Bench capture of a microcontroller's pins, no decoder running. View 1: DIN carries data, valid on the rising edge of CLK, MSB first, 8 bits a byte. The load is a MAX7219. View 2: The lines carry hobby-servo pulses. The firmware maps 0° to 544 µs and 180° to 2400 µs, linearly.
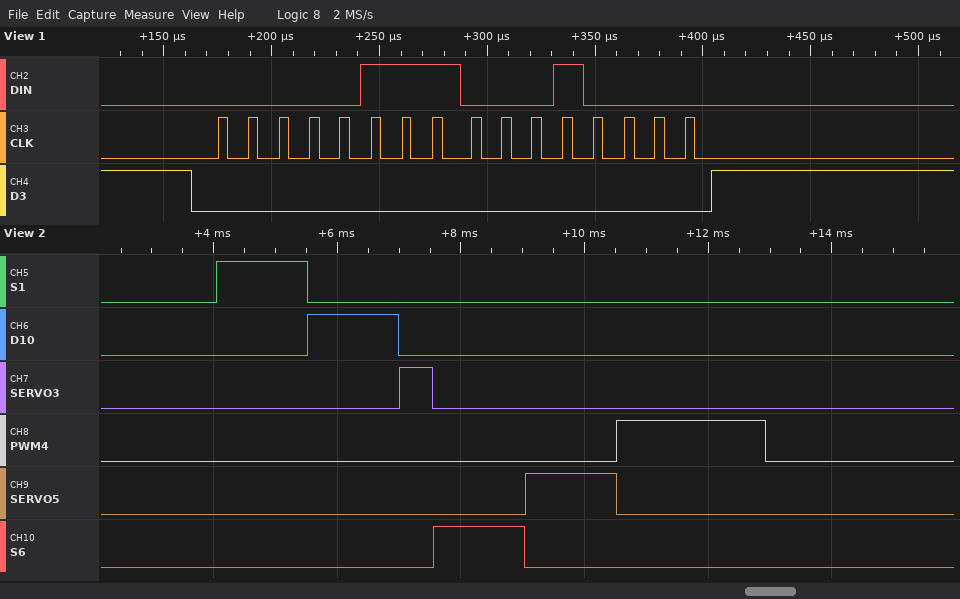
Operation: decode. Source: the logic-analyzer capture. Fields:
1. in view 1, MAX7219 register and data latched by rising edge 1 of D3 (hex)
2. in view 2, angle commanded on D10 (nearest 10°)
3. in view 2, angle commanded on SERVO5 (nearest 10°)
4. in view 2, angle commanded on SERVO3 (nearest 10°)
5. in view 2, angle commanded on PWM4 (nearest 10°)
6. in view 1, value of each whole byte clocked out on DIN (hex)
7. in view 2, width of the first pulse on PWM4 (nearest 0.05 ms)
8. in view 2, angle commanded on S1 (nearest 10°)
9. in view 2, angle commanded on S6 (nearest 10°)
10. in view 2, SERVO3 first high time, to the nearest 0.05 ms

register 0x7, data 0x10
90°
90°
0°
180°
0x07 0x10
2.40 ms
90°
90°
0.55 ms
